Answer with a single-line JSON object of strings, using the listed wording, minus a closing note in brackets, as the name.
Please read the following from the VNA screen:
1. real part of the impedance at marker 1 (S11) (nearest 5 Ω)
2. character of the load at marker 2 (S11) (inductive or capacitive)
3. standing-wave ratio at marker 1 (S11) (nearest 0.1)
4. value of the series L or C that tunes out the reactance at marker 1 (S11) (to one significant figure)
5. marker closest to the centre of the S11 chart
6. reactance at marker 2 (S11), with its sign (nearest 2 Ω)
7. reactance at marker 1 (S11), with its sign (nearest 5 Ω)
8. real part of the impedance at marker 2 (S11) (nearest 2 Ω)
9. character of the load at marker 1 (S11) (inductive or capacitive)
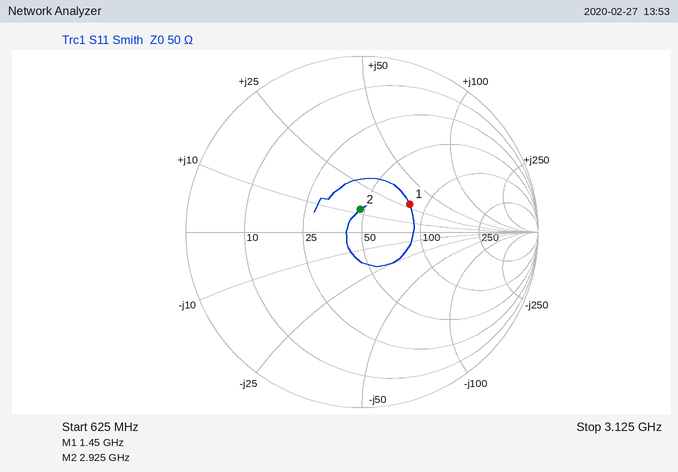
{"real part of the impedance at marker 1 (S11)": "80 Ω", "character of the load at marker 2 (S11)": "inductive", "standing-wave ratio at marker 1 (S11)": "1.9", "value of the series L or C that tunes out the reactance at marker 1 (S11)": "4 pF", "marker closest to the centre of the S11 chart": "marker 2", "reactance at marker 2 (S11), with its sign": "+12 Ω", "reactance at marker 1 (S11), with its sign": "+30 Ω", "real part of the impedance at marker 2 (S11)": "48 Ω", "character of the load at marker 1 (S11)": "inductive"}
